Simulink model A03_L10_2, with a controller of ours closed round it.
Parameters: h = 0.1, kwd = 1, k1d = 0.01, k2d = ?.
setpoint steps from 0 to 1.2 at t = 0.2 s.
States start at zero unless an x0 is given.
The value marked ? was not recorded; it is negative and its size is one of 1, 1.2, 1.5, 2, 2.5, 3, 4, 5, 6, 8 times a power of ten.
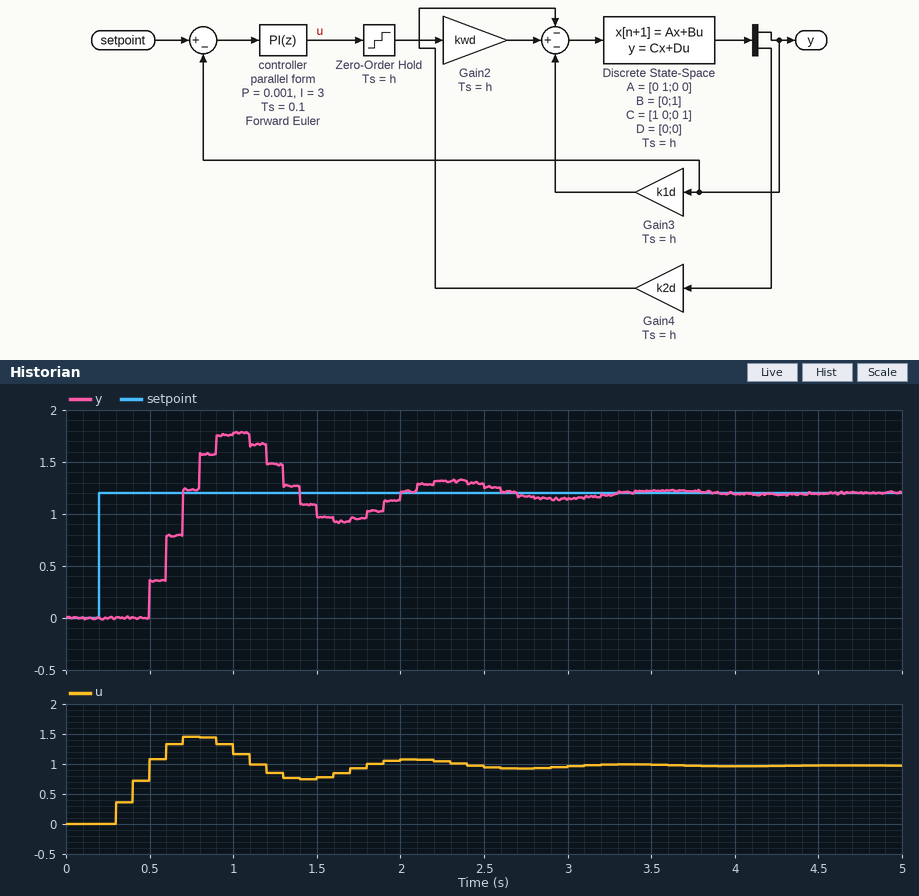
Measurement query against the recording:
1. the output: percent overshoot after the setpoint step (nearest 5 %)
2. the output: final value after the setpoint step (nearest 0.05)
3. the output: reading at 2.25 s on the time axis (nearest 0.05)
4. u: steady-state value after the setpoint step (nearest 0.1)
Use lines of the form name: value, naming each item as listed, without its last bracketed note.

the output: percent overshoot after the setpoint step: 50 %
the output: final value after the setpoint step: 1.20
the output: reading at 2.25 s on the time axis: 1.30
u: steady-state value after the setpoint step: 1.0
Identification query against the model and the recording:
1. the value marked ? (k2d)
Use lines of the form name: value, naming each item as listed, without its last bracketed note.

the value marked ?: -0.2
